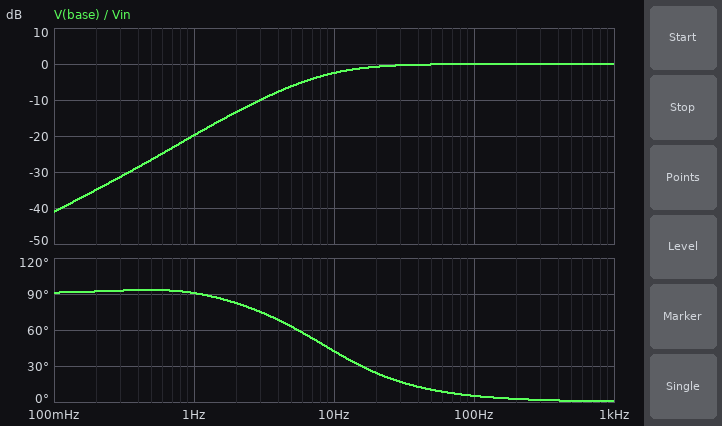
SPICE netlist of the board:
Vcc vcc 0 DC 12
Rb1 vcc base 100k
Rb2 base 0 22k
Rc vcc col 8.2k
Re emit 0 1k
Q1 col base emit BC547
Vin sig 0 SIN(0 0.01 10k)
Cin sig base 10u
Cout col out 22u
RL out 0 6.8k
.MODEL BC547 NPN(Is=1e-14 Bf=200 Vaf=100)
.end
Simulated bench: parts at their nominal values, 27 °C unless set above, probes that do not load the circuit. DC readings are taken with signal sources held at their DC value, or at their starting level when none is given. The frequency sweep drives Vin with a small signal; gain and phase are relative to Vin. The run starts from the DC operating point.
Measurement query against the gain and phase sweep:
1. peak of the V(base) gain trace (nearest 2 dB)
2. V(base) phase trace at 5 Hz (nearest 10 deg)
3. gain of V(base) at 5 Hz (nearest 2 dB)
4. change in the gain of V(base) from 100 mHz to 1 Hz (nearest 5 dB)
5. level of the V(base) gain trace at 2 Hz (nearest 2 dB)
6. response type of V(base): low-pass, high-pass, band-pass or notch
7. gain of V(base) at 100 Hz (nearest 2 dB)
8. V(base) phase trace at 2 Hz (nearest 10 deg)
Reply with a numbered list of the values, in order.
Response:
1. 0 dB
2. 60 deg
3. -6 dB
4. 20 dB
5. -14 dB
6. high-pass
7. 0 dB
8. 80 deg
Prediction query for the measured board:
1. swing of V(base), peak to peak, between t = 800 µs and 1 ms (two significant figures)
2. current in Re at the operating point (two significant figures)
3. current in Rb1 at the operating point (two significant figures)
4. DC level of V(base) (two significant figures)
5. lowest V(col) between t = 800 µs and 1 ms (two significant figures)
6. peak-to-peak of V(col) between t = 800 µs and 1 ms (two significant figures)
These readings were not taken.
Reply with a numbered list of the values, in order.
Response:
1. 20 mV
2. 1.3 mA
3. 100 µA
4. 2.0 V
5. 1.4 V
6. 35 mV
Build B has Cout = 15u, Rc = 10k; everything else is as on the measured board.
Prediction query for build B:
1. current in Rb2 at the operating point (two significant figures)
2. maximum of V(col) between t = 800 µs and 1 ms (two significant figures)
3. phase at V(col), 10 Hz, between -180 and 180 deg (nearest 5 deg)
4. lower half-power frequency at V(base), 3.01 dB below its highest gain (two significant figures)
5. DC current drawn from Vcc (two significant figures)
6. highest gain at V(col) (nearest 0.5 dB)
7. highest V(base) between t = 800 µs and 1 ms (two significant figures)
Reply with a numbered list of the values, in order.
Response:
1. 80 µA
2. 1.2 V
3. -125 deg
4. 15 Hz
5. 1.2 mA
6. -9.5 dB
7. 1.8 V
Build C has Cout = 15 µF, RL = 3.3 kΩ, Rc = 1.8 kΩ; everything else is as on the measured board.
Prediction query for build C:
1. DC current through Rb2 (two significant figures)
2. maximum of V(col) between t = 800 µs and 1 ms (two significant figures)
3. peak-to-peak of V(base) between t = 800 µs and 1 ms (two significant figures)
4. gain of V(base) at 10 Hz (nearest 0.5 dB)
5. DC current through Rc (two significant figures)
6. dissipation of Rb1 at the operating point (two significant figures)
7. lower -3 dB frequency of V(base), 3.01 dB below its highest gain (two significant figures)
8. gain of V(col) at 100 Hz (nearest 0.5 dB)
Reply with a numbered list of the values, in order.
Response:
1. 93 µA
2. 9.5 V
3. 20 mV
4. 0 dB
5. 1.4 mA
6. 990 µW
7. 960 mHz
8. 1.0 dB
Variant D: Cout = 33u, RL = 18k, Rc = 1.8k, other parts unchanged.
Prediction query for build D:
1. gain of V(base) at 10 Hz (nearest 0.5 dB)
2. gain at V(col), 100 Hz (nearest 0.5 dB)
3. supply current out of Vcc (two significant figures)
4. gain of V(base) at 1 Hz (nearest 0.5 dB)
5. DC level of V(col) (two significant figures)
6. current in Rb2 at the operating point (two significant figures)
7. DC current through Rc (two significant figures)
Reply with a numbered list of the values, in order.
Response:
1. 0 dB
2. 4.0 dB
3. 1.5 mA
4. -3.0 dB
5. 9.5 V
6. 93 µA
7. 1.4 mA
